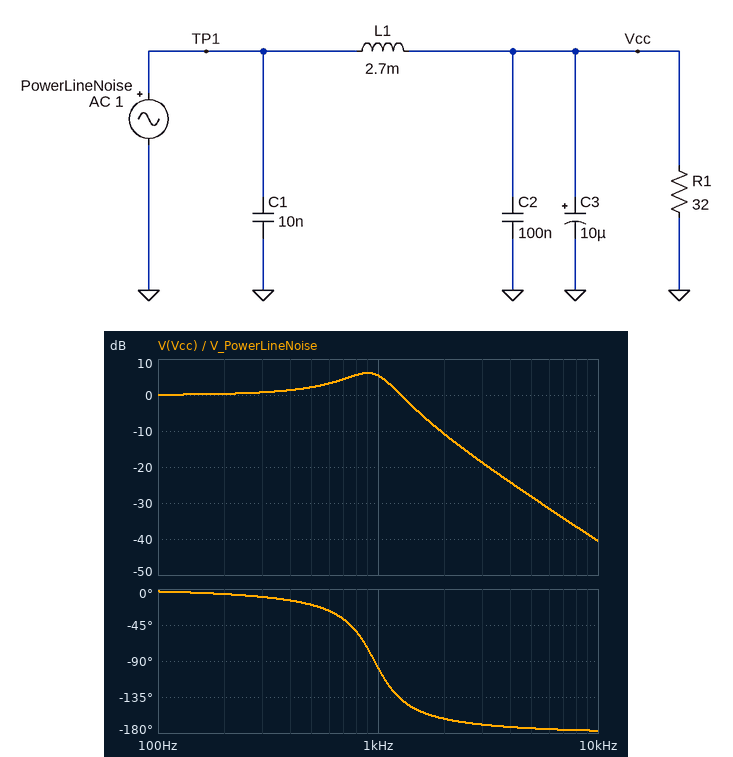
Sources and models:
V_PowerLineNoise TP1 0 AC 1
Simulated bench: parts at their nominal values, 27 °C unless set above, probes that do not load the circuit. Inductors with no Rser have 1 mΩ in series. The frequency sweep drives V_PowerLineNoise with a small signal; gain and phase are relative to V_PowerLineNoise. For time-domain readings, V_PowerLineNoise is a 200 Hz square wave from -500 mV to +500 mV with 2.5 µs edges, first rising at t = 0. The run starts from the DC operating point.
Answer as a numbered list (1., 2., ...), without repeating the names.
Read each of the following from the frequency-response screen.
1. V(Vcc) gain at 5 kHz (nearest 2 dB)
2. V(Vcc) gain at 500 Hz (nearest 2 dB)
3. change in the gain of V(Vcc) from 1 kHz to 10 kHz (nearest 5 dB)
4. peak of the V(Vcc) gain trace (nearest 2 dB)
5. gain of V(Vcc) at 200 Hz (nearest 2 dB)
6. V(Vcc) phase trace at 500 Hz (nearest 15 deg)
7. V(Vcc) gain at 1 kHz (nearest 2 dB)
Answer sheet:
1. -28 dB
2. 2 dB
3. -45 dB
4. 6 dB
5. 0 dB
6. -15 deg
7. 6 dB
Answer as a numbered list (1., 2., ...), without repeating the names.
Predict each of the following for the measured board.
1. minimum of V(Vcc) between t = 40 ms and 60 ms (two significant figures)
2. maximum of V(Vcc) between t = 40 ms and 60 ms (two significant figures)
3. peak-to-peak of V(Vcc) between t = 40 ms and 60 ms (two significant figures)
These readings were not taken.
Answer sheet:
1. -940 mV
2. 940 mV
3. 1.9 V
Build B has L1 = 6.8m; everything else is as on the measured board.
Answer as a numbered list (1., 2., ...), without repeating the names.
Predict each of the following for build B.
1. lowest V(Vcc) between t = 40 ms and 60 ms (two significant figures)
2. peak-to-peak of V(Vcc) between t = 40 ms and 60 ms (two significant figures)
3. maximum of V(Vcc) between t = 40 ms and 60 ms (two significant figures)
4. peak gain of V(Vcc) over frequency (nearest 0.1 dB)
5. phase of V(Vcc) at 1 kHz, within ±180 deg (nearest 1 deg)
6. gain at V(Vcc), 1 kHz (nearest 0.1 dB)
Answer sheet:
1. -750 mV
2. 1.5 V
3. 750 mV
4. 2.6 dB
5. -142 deg
6. -6.7 dB
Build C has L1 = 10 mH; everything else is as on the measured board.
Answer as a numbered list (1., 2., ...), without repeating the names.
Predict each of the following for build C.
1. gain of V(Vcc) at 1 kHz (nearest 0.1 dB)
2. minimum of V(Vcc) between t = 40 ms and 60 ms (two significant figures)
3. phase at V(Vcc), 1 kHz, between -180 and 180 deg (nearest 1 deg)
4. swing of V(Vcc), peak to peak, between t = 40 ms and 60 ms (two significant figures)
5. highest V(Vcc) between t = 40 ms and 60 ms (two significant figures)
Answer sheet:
1. -11.1 dB
2. -670 mV
3. -147 deg
4. 1.3 V
5. 670 mV
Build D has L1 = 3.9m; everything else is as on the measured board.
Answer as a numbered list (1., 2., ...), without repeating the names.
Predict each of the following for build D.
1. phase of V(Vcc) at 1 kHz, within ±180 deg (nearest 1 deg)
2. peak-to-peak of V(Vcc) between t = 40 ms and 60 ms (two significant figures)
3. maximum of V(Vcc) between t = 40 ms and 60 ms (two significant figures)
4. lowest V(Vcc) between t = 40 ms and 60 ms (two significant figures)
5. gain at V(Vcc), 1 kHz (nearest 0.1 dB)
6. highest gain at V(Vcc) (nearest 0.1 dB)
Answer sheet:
1. -126 deg
2. 1.7 V
3. 860 mV
4. -860 mV
5. 0.5 dB
6. 4.7 dB
